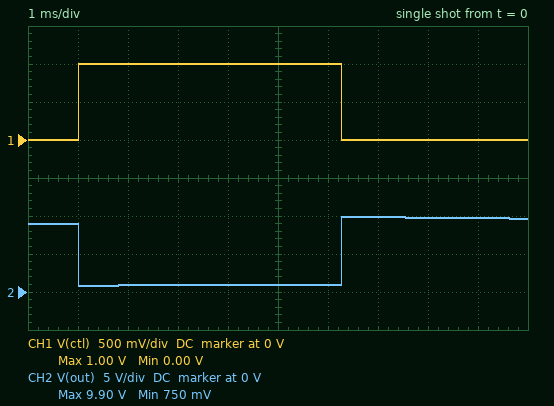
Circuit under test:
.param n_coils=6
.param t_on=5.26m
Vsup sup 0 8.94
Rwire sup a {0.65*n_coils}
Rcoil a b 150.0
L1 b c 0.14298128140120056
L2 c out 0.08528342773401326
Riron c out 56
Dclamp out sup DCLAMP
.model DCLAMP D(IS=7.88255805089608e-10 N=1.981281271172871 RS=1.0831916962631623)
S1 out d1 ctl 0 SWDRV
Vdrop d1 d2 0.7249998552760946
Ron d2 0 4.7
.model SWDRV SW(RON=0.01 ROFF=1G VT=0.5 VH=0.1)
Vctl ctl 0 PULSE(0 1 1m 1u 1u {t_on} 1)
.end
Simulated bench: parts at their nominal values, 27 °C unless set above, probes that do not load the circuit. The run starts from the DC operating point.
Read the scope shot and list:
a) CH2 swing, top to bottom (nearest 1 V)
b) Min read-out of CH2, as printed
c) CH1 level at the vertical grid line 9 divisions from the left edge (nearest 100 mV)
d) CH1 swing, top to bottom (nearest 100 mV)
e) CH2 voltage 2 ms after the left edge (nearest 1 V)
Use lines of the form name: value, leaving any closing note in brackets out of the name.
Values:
CH2 swing, top to bottom: 9 V
Min read-out of CH2, as printed: 750 mV
CH1 level at the vertical grid line 9 divisions from the left edge: 0 V
CH1 swing, top to bottom: 1.0 V
CH2 voltage 2 ms after the left edge: 1 V
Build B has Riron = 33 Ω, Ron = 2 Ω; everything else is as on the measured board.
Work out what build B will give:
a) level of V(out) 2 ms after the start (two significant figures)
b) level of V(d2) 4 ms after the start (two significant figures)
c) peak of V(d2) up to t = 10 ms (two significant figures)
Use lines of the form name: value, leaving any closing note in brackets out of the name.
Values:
level of V(out) 2 ms after the start: 790 mV
level of V(d2) 4 ms after the start: 92 mV
peak of V(d2) up to t = 10 ms: 99 mV
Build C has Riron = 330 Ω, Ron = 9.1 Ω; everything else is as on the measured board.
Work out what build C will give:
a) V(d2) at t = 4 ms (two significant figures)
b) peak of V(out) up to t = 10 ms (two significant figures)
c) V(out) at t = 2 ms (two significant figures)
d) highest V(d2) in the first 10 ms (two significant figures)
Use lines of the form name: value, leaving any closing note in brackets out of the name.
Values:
V(d2) at t = 4 ms: 400 mV
peak of V(out) up to t = 10 ms: 9.9 V
V(out) at t = 2 ms: 970 mV
highest V(d2) in the first 10 ms: 450 mV
